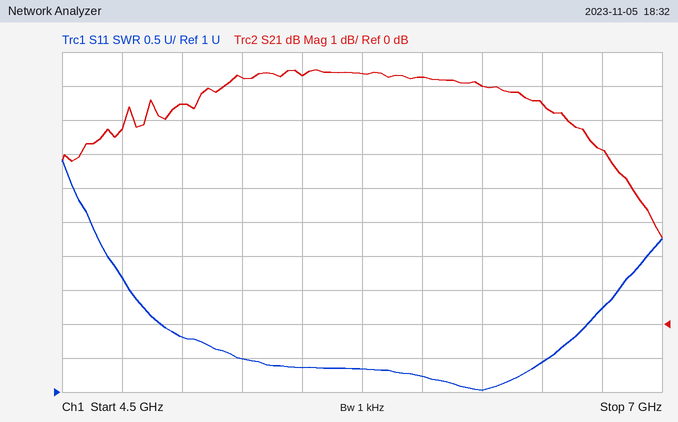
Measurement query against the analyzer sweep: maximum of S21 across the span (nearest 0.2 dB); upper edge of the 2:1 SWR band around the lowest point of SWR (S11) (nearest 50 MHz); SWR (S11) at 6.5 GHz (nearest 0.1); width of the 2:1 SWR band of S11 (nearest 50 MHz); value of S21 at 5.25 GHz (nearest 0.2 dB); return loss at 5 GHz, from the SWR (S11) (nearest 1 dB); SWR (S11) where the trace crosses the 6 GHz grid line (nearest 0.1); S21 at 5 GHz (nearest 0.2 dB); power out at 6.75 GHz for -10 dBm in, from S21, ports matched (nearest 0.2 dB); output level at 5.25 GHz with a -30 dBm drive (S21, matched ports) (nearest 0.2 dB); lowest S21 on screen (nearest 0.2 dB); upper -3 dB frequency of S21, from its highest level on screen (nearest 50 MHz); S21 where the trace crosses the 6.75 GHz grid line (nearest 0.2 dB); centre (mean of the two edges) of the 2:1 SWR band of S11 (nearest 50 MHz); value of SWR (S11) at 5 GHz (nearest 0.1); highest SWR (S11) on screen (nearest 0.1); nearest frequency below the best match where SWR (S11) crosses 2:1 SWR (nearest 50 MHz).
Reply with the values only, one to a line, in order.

7.4 dB
6.70 GHz
1.4
1.80 GHz
7.2 dB
11 dB
1.2
6.4 dB
-4.8 dBm
-22.8 dBm
2.6 dB
6.80 GHz
5.2 dB
5.80 GHz
1.8
4.4
4.90 GHz
